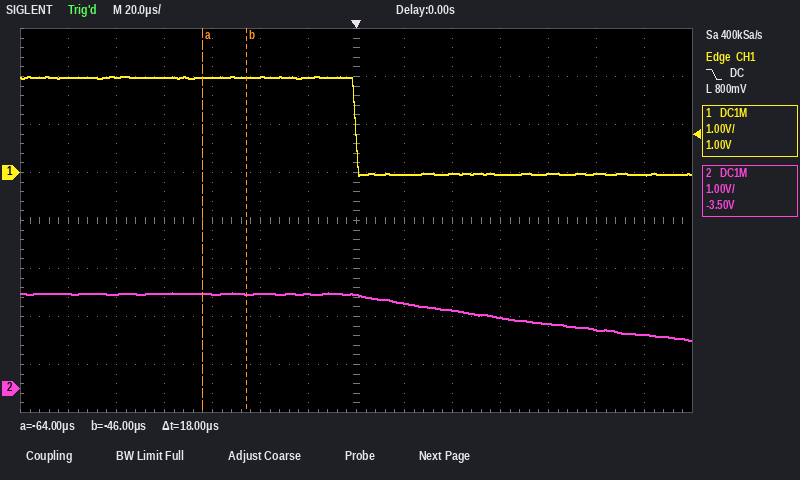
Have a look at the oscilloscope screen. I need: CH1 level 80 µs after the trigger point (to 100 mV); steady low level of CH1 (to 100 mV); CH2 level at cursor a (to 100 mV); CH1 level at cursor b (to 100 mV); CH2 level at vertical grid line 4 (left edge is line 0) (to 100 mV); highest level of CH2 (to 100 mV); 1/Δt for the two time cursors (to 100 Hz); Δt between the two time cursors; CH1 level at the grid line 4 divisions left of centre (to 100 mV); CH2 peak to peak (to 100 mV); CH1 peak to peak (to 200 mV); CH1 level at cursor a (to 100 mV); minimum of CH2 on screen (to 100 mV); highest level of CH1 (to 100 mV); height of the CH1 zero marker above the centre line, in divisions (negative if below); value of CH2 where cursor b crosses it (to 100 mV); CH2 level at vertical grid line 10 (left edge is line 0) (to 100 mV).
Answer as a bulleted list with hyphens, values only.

- 0.0 V
- 0.0 V
- 2.0 V
- 2.0 V
- 2.0 V
- 2.0 V
- 55.6 kHz
- 18 µs
- 2.0 V
- 1.0 V
- 2.0 V
- 2.0 V
- 1.0 V
- 2.0 V
- +1.0 div
- 2.0 V
- 1.5 V
